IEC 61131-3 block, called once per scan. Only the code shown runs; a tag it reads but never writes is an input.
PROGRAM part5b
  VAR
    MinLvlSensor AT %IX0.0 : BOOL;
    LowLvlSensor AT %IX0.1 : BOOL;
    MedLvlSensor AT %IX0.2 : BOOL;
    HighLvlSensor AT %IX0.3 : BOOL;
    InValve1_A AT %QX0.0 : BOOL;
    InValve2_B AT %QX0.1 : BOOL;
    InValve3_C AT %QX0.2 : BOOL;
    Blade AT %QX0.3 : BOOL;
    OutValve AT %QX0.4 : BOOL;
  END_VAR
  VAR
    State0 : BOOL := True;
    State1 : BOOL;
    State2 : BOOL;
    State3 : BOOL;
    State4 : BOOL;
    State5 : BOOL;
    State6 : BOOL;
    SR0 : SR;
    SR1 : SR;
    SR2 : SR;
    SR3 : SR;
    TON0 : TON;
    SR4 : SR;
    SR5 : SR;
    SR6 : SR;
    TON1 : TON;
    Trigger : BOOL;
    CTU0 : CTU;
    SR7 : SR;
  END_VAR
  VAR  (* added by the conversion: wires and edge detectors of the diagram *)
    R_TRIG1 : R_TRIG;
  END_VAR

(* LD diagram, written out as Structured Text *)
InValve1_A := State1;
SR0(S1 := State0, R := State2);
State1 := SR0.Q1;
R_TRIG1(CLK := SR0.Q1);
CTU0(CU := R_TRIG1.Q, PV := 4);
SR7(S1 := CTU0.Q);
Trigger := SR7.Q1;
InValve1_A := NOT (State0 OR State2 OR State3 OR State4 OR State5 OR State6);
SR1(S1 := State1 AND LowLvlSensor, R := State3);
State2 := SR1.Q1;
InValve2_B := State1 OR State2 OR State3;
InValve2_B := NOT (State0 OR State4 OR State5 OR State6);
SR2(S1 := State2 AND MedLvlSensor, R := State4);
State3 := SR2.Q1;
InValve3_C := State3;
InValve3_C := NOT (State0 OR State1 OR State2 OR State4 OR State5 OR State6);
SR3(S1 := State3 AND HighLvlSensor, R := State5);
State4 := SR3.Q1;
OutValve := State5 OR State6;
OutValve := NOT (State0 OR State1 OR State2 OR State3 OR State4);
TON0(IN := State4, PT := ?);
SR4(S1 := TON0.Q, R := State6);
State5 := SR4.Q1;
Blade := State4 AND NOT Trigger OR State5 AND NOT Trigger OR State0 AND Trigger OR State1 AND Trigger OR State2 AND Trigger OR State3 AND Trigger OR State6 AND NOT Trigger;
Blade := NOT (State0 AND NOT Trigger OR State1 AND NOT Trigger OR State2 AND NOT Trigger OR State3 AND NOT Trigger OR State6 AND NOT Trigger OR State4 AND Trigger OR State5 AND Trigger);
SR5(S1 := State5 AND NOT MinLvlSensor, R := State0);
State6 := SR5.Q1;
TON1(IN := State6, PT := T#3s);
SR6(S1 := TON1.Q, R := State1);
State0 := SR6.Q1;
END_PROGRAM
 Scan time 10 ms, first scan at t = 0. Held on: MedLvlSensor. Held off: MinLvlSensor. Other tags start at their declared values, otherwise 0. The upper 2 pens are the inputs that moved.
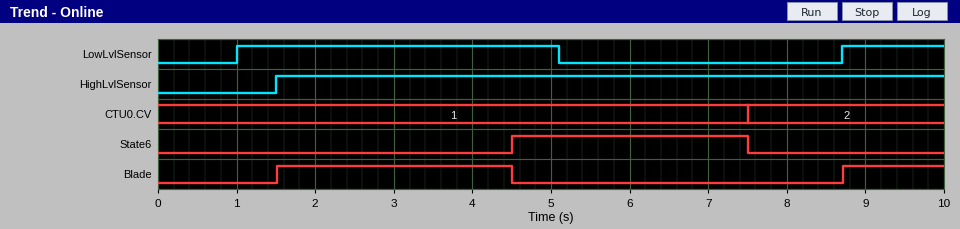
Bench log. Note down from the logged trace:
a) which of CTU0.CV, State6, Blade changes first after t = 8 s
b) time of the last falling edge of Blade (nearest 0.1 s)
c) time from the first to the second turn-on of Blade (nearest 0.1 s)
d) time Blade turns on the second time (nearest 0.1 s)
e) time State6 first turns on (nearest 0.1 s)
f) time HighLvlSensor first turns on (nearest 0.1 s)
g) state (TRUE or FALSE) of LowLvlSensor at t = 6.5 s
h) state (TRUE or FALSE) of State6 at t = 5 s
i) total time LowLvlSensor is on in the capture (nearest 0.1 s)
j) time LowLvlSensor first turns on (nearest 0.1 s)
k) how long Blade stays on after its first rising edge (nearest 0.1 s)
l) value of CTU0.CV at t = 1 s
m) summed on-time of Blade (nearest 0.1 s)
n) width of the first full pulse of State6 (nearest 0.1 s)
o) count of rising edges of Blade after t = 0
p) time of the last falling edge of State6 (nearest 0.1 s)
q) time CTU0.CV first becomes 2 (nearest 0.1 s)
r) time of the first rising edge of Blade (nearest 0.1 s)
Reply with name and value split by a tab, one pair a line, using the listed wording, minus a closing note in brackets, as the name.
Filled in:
which of CTU0.CV, State6, Blade changes first after t = 8 s	Blade
time of the last falling edge of Blade	4.5 s
time from the first to the second turn-on of Blade	7.2 s
time Blade turns on the second time	8.7 s
time State6 first turns on	4.5 s
time HighLvlSensor first turns on	1.5 s
state (TRUE or FALSE) of LowLvlSensor at t = 6.5 s	FALSE
state (TRUE or FALSE) of State6 at t = 5 s	TRUE
total time LowLvlSensor is on in the capture	5.4 s
time LowLvlSensor first turns on	1.0 s
how long Blade stays on after its first rising edge	3.0 s
value of CTU0.CV at t = 1 s	1
summed on-time of Blade	4.3 s
width of the first full pulse of State6	3.0 s
count of rising edges of Blade after t = 0	2
time of the last falling edge of State6	7.5 s
time CTU0.CV first becomes 2	7.5 s
time of the first rising edge of Blade	1.5 s
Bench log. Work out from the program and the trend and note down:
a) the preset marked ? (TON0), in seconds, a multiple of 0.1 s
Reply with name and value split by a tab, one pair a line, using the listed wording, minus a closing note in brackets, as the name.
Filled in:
the preset marked ? (TON0), in seconds, a multiple of 0.1 s	3.0 s
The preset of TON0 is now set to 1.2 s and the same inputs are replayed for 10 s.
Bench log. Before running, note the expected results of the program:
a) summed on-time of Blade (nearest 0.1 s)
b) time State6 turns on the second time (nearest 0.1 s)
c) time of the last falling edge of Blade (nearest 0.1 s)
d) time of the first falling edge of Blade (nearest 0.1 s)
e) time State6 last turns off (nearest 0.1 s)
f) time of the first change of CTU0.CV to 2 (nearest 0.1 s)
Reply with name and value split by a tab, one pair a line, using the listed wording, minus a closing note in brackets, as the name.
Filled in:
summed on-time of Blade	2.4 s
time State6 turns on the second time	9.9 s
time of the last falling edge of Blade	9.9 s
time of the first falling edge of Blade	2.7 s
time State6 last turns off	5.7 s
time of the first change of CTU0.CV to 2	5.7 s
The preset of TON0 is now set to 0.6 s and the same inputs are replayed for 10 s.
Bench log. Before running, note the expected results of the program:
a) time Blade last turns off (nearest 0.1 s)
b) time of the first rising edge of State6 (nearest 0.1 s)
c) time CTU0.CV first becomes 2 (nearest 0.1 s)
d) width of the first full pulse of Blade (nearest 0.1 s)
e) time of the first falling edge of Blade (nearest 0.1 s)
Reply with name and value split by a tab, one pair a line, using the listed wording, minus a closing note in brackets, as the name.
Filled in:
time Blade last turns off	9.3 s
time of the first rising edge of State6	2.1 s
time CTU0.CV first becomes 2	5.1 s
width of the first full pulse of Blade	0.6 s
time of the first falling edge of Blade	2.1 s
